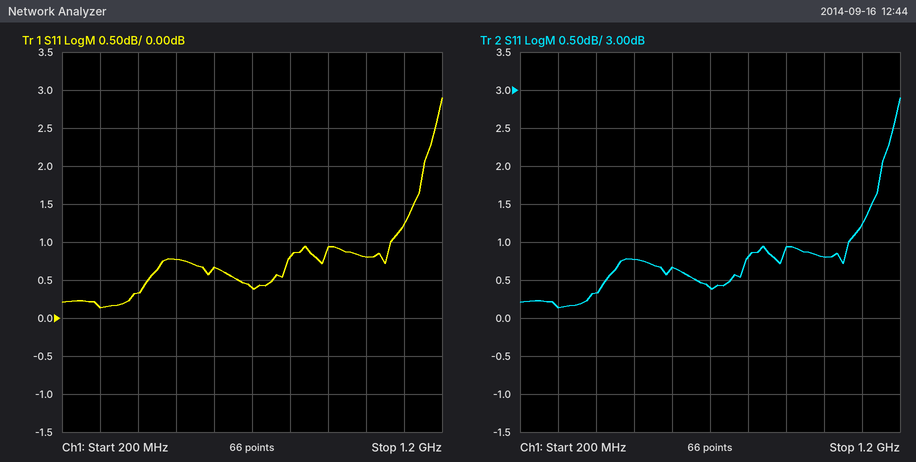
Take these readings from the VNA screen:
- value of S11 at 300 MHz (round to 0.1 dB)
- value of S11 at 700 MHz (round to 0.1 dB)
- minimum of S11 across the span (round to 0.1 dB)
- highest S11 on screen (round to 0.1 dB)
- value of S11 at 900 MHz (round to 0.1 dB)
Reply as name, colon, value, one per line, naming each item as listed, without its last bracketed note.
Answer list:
value of S11 at 300 MHz: 0.1 dB
value of S11 at 700 MHz: 0.4 dB
minimum of S11 across the span: 0.1 dB
highest S11 on screen: 2.9 dB
value of S11 at 900 MHz: 0.9 dB
